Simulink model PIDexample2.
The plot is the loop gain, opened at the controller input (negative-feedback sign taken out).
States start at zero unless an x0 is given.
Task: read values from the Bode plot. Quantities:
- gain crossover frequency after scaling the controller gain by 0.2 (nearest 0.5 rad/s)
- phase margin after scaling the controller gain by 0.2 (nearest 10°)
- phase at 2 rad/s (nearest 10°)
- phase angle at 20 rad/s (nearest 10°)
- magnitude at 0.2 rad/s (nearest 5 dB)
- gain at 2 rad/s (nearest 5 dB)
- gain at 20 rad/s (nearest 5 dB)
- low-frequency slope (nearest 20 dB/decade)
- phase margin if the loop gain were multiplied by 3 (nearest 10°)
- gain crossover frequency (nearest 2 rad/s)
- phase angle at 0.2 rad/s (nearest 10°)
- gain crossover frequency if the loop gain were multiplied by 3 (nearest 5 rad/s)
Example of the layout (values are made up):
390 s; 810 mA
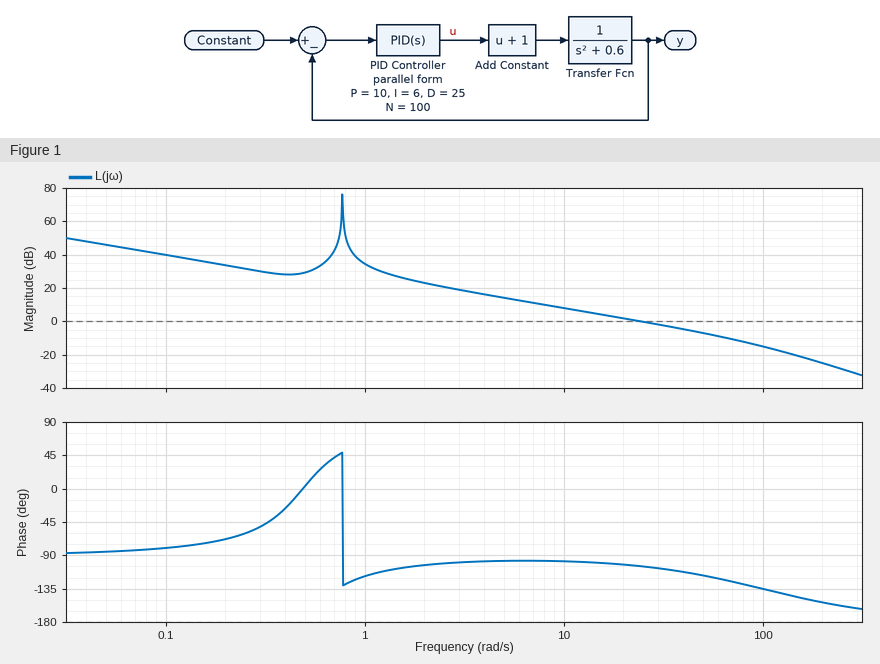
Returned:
5.0 rad/s; 80°; -100°; -100°; 35 dB; 25 dB; 0 dB; -20 dB/decade; 60°; 24 rad/s; -70°; 65 rad/s
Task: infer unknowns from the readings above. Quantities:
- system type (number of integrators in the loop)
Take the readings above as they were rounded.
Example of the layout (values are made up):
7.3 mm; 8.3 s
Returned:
1
